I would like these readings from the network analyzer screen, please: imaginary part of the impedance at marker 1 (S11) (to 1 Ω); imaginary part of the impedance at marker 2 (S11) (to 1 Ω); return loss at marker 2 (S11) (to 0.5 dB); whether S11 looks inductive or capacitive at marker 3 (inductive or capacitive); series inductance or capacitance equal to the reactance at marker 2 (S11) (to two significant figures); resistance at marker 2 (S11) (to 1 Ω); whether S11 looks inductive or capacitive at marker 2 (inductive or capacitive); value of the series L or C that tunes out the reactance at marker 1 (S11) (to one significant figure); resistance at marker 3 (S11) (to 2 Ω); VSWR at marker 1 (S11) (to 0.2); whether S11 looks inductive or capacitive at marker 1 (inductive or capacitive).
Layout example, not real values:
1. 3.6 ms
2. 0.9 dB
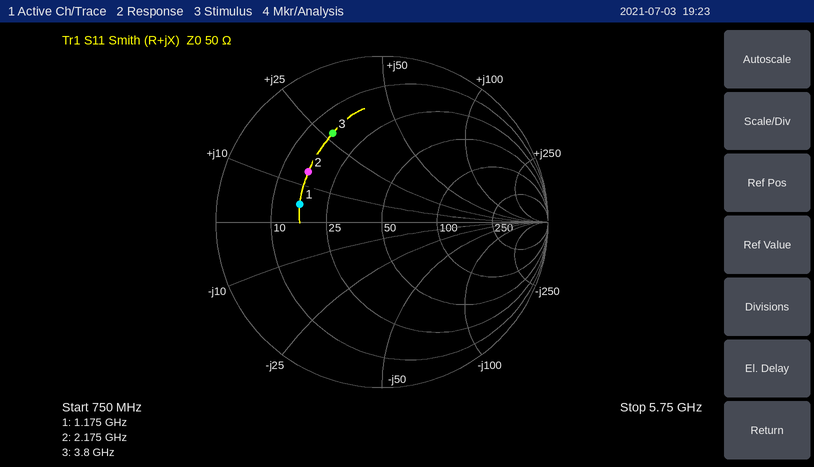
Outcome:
1. +5 Ω
2. +14 Ω
3. 5.5 dB
4. inductive
5. 1.0 nH
6. 16 Ω
7. inductive
8. 30 pF
9. 16 Ω
10. 3.0
11. inductive
